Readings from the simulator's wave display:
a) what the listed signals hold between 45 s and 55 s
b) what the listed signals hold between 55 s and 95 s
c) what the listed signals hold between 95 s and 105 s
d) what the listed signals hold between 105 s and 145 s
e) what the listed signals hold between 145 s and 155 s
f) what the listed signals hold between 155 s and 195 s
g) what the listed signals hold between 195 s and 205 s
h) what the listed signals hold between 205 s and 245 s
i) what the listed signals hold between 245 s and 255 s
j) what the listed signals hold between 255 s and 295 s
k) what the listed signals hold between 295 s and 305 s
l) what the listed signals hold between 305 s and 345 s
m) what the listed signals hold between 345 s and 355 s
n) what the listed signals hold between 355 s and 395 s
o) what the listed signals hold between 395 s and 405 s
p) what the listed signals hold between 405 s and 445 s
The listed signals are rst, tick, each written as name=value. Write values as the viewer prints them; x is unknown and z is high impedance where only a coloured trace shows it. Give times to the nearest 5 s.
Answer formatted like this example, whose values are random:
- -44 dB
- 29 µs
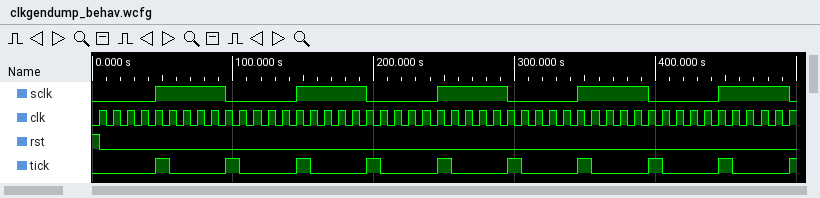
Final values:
- rst=0, tick=1
- rst=0, tick=0
- rst=0, tick=1
- rst=0, tick=0
- rst=0, tick=1
- rst=0, tick=0
- rst=0, tick=1
- rst=0, tick=0
- rst=0, tick=1
- rst=0, tick=0
- rst=0, tick=1
- rst=0, tick=0
- rst=0, tick=1
- rst=0, tick=0
- rst=0, tick=1
- rst=0, tick=0
